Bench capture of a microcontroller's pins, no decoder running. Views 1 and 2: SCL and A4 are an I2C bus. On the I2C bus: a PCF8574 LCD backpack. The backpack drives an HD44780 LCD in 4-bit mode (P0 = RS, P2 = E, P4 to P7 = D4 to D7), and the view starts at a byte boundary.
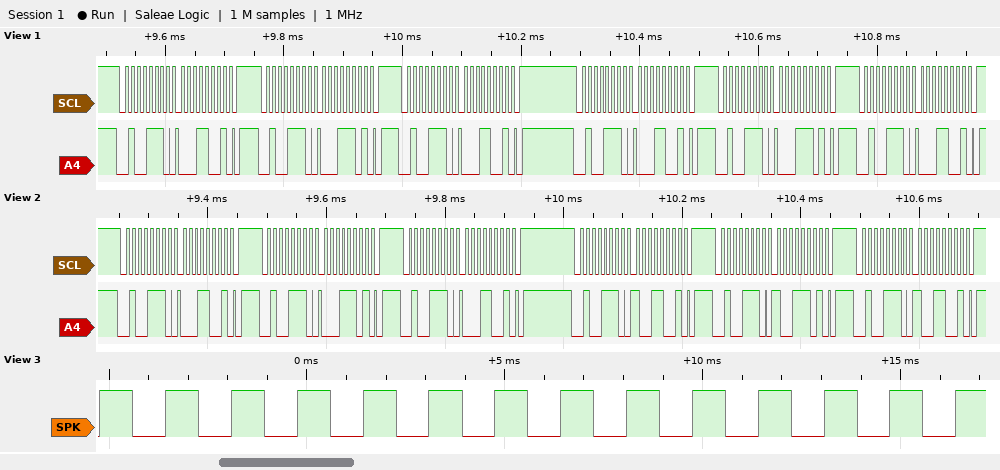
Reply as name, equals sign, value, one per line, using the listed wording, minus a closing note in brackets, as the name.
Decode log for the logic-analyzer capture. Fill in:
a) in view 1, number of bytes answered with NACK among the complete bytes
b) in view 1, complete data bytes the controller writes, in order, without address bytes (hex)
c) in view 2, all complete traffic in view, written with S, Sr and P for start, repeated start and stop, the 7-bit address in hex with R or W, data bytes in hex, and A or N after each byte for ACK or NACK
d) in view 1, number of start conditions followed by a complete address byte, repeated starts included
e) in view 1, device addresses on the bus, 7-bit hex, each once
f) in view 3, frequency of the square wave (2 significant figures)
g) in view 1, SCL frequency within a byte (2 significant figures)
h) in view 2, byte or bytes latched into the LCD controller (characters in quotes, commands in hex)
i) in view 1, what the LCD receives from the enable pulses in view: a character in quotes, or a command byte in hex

in view 1, number of bytes answered with NACK among the complete bytes = 0
in view 1, complete data bytes the controller writes, in order, without address bytes = 19 1D 19 19 1D 19
in view 2, all complete traffic in view, written with S, Sr and P for start, repeated start and stop, the 7-bit address in hex with R or W, data bytes in hex, and A or N after each byte for ACK or NACK = S 27W A 19 A P S 27W A 1D A P S 27W A 19 A P S 27W A 99 A P S 27W A 9D A P S 27W A 99 A P
in view 1, number of start conditions followed by a complete address byte, repeated starts included = 6
in view 1, device addresses on the bus, 7-bit hex, each once = 0x27
in view 3, frequency of the square wave = 600 Hz
in view 1, SCL frequency within a byte = 100 kHz
in view 2, byte or bytes latched into the LCD controller = data 0x19
in view 1, what the LCD receives from the enable pulses in view: a character in quotes, or a command byte in hex = data 0x11
